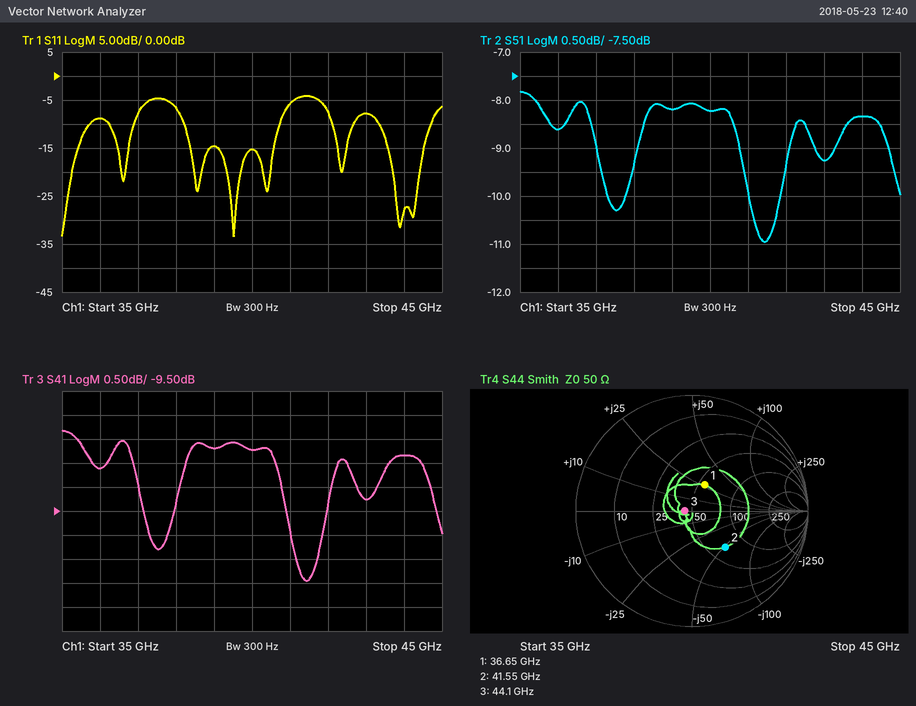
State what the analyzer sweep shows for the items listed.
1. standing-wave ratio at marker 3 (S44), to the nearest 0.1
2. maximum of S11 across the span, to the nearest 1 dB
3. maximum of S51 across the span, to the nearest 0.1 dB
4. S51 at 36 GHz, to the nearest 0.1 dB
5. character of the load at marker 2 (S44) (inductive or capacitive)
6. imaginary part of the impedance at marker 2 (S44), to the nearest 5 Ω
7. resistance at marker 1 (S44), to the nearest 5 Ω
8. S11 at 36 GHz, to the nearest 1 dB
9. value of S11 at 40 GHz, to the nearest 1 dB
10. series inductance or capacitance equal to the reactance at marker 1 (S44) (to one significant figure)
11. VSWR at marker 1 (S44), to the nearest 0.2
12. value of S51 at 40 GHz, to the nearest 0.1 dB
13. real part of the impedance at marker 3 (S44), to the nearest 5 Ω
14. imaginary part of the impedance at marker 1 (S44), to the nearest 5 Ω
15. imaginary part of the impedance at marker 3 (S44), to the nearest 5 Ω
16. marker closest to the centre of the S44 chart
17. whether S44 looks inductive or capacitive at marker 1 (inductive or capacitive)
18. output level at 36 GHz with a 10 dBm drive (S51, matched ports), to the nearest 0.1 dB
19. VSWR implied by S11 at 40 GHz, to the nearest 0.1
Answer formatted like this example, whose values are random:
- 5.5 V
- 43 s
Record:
- 1.1
- -4 dB
- -7.8 dB
- -8.6 dB
- capacitive
- -50 Ω
- 55 Ω
- -9 dB
- -15 dB
- 100 pH
- 1.6
- -8.2 dB
- 45 Ω
- +25 Ω
- 0 Ω
- marker 3
- inductive
- 1.4 dBm
- 1.4
